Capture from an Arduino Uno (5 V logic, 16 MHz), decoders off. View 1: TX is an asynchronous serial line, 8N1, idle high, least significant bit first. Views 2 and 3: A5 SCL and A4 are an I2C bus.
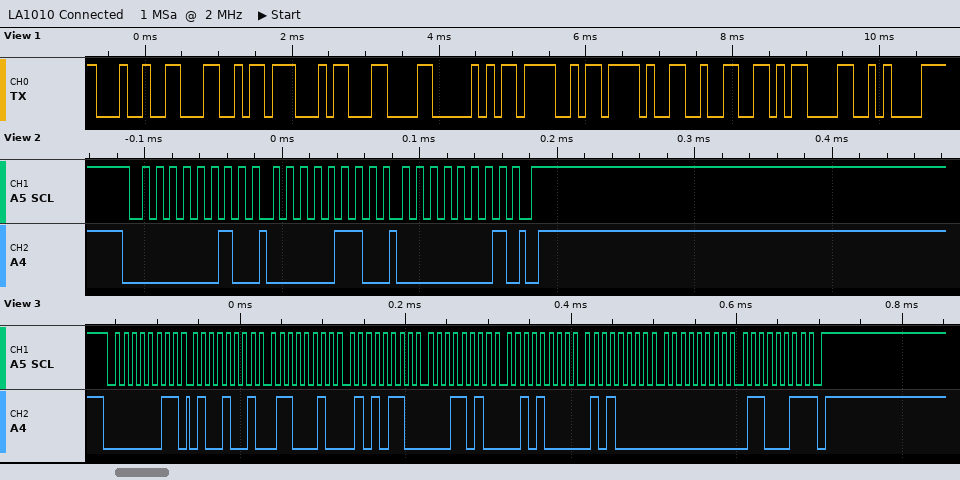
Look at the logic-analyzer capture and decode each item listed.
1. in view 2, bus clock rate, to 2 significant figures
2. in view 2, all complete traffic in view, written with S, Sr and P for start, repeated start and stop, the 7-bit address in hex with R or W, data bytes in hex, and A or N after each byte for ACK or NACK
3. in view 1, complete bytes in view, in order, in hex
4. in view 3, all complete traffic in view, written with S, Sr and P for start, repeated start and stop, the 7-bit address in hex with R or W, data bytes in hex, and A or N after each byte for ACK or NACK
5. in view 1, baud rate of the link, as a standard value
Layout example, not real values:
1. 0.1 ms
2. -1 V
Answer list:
1. 100 kHz
2. S 01W A 06 A 01 A P
3. 24 4C 47 0C 50 4F 2F 32 0D 0A
4. S 01R A 49 A 62 A 56 A 1A A 28 A 50 A 00 A 63 N P
5. 9600 baud
